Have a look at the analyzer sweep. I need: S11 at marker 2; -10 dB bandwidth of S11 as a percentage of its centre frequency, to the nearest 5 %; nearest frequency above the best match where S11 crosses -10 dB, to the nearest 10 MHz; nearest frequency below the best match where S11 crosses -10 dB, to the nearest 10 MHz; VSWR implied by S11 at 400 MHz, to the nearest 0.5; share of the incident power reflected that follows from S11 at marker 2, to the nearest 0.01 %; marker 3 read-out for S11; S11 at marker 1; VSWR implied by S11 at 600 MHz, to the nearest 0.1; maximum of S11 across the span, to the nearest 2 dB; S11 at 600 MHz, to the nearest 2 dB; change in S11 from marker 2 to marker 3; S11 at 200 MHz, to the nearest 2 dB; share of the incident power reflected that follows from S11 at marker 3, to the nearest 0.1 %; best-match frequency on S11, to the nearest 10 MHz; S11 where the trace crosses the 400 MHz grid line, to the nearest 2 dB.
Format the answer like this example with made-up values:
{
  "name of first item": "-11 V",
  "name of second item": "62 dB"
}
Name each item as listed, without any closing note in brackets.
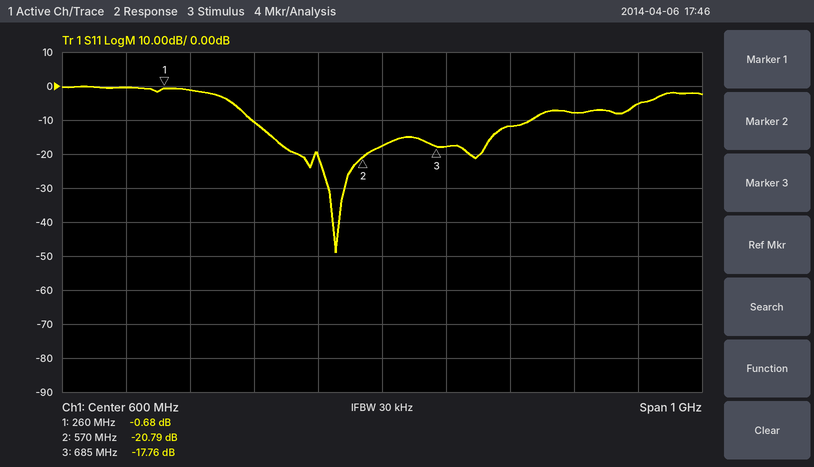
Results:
{
  "S11 at marker 2": "-20.79 dB",
  "-10 dB bandwidth of S11 as a percentage of its centre frequency, to the nearest 5 %": "70 %",
  "nearest frequency above the best match where S11 crosses -10 dB, to the nearest 10 MHz": "830 MHz",
  "nearest frequency below the best match where S11 crosses -10 dB, to the nearest 10 MHz": "400 MHz",
  "VSWR implied by S11 at 400 MHz, to the nearest 0.5": "2.0",
  "share of the incident power reflected that follows from S11 at marker 2, to the nearest 0.01 %": "0.83 %",
  "marker 3 read-out for S11": "-17.76 dB",
  "S11 at marker 1": "-0.68 dB",
  "VSWR implied by S11 at 600 MHz, to the nearest 0.1": "1.3",
  "maximum of S11 across the span, to the nearest 2 dB": "0 dB",
  "S11 at 600 MHz, to the nearest 2 dB": "-18 dB",
  "change in S11 from marker 2 to marker 3": "3.03 dB",
  "S11 at 200 MHz, to the nearest 2 dB": "0 dB",
  "share of the incident power reflected that follows from S11 at marker 3, to the nearest 0.1 %": "1.7 %",
  "best-match frequency on S11, to the nearest 10 MHz": "530 MHz",
  "S11 where the trace crosses the 400 MHz grid line, to the nearest 2 dB": "-10 dB"
}
